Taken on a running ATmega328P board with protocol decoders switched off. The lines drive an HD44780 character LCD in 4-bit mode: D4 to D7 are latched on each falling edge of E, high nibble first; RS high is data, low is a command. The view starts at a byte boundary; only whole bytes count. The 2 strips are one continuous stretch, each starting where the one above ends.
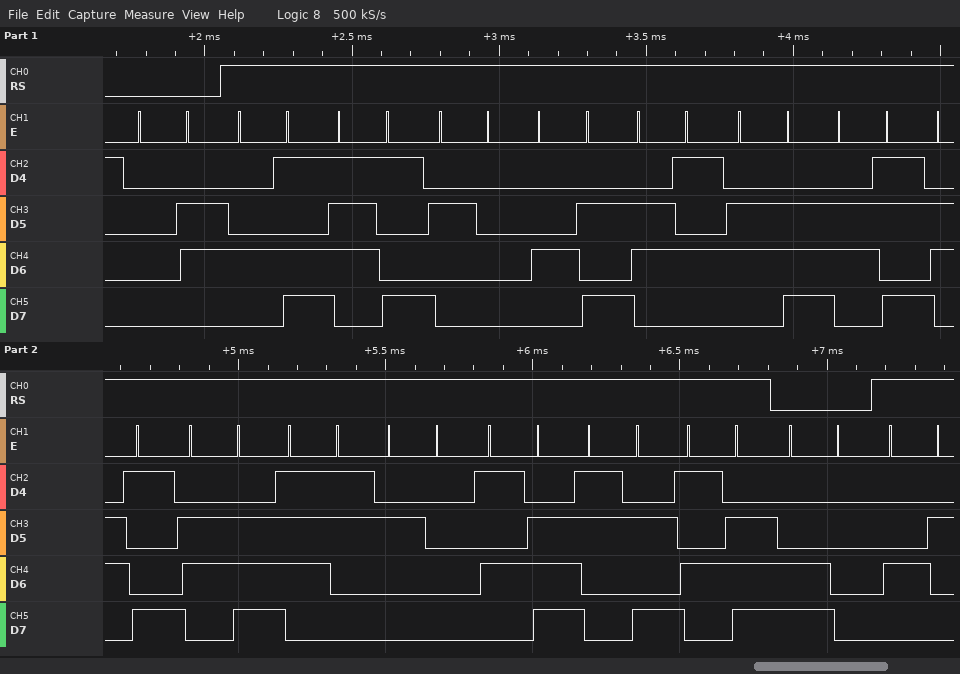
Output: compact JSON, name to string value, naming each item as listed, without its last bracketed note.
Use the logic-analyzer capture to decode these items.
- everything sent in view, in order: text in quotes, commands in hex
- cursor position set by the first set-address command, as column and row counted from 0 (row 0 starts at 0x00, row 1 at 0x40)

{"everything sent in view, in order: text in quotes, commands in hex": "0x06 \"My Jenkins ^:^\" 0xC0 \"B\"", "cursor position set by the first set-address command, as column and row counted from 0": "column 0, row 1"}
